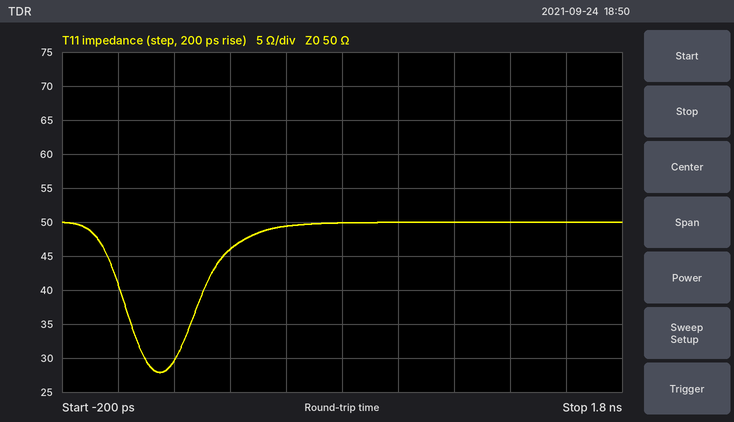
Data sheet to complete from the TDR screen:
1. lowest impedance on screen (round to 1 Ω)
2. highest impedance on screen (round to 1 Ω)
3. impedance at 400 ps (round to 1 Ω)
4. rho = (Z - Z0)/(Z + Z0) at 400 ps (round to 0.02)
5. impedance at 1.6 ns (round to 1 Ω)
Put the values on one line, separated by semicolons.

28 Ω; 50 Ω; 46 Ω; -0.04; 50 Ω
